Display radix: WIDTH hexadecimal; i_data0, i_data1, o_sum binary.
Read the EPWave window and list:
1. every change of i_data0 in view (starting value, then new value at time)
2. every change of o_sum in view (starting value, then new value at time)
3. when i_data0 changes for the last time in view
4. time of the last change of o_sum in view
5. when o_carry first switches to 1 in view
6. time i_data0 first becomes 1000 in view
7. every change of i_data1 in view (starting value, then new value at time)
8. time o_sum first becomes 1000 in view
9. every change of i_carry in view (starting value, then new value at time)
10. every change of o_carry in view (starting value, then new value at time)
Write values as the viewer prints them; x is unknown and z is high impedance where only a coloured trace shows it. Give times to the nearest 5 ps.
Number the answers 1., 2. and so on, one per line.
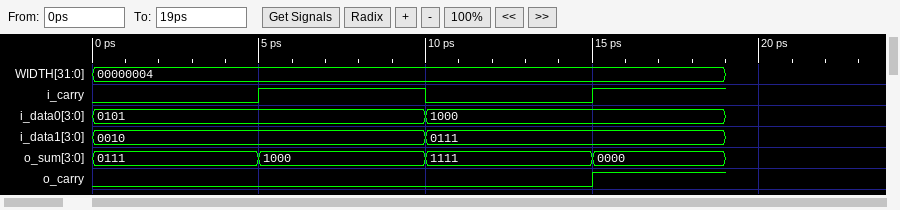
1. 0101, 1000 at 10 ps
2. 0111, 1000 at 5 ps, 1111 at 10 ps, 0000 at 15 ps
3. 10 ps
4. 15 ps
5. 15 ps
6. 10 ps
7. 0010, 0111 at 10 ps
8. 5 ps
9. 0, 1 at 5 ps, 0 at 10 ps, 1 at 15 ps
10. 0, 1 at 15 ps
